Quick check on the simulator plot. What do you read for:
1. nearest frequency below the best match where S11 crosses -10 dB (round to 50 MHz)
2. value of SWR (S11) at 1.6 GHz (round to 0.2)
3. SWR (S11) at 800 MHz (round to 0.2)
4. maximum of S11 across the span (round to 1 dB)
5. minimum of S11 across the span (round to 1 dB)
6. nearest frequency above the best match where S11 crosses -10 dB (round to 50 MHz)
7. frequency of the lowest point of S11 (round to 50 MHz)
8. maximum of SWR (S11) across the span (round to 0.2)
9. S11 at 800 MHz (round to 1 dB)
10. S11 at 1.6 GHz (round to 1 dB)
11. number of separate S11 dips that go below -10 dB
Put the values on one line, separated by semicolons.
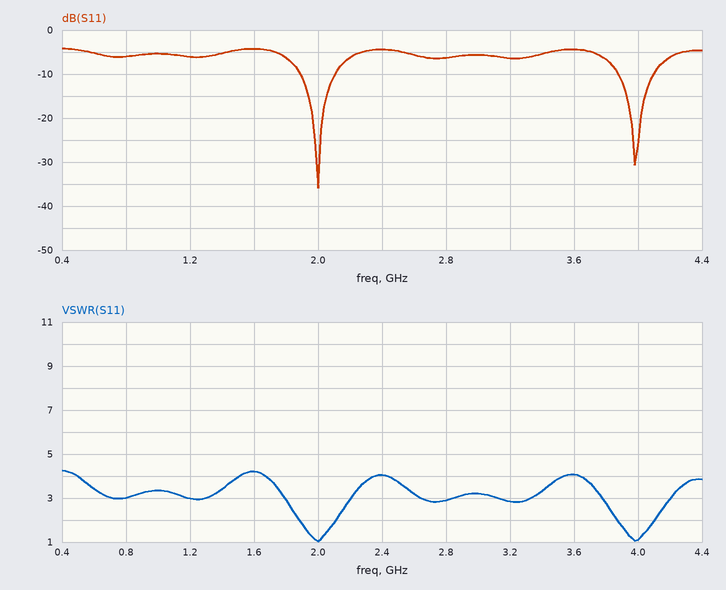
1.90 GHz; 4.2; 3.0; -4 dB; -36 dB; 2.10 GHz; 2.00 GHz; 4.2; -6 dB; -4 dB; 2
